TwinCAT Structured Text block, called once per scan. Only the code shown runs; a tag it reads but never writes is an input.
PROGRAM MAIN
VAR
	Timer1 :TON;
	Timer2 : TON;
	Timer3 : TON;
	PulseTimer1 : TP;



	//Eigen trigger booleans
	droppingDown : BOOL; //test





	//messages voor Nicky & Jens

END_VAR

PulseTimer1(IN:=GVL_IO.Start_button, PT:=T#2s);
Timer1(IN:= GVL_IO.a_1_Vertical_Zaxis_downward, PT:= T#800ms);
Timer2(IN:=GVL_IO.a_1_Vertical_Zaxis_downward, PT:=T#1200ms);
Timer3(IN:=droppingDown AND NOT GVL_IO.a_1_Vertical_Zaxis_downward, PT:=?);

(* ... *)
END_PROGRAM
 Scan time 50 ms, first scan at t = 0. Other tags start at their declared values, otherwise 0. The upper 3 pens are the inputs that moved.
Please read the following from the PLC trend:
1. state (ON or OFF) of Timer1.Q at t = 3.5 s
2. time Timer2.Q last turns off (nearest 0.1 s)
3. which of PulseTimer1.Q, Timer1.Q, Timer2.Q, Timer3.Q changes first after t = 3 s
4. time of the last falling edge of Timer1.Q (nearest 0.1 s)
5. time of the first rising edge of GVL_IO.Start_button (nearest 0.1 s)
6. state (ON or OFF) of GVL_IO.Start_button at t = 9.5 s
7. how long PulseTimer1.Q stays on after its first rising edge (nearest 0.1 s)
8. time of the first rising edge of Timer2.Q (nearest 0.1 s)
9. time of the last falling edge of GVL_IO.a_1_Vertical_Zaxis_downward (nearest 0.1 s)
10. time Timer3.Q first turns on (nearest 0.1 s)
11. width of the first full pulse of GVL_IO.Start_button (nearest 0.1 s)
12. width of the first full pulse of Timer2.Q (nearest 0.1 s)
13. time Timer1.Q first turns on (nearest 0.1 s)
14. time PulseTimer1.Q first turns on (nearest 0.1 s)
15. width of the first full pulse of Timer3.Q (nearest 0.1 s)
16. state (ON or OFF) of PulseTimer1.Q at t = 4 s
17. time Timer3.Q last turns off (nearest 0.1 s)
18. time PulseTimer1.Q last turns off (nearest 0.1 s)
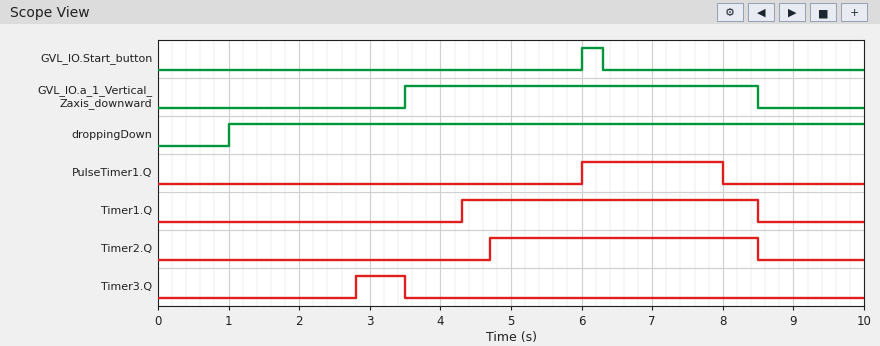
OFF
8.5 s
Timer3.Q
8.5 s
6.0 s
OFF
2.0 s
4.7 s
8.5 s
2.8 s
0.3 s
3.8 s
4.3 s
6.0 s
0.7 s
OFF
3.5 s
8.0 s
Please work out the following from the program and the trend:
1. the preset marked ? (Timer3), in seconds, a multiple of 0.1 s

1.8 s
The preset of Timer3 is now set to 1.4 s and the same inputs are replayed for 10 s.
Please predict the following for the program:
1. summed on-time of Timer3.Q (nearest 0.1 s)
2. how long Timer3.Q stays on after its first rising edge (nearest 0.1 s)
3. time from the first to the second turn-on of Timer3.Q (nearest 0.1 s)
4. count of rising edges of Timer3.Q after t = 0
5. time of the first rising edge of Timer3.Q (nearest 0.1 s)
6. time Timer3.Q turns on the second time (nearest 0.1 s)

1.2 s
1.1 s
7.5 s
2
2.4 s
9.9 s
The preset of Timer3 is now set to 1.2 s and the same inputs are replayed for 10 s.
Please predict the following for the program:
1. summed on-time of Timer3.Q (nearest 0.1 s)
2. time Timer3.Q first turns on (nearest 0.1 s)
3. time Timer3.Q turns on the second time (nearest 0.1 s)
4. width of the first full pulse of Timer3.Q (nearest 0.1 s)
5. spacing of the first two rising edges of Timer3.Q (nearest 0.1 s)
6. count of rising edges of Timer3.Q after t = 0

1.6 s
2.2 s
9.7 s
1.3 s
7.5 s
2
